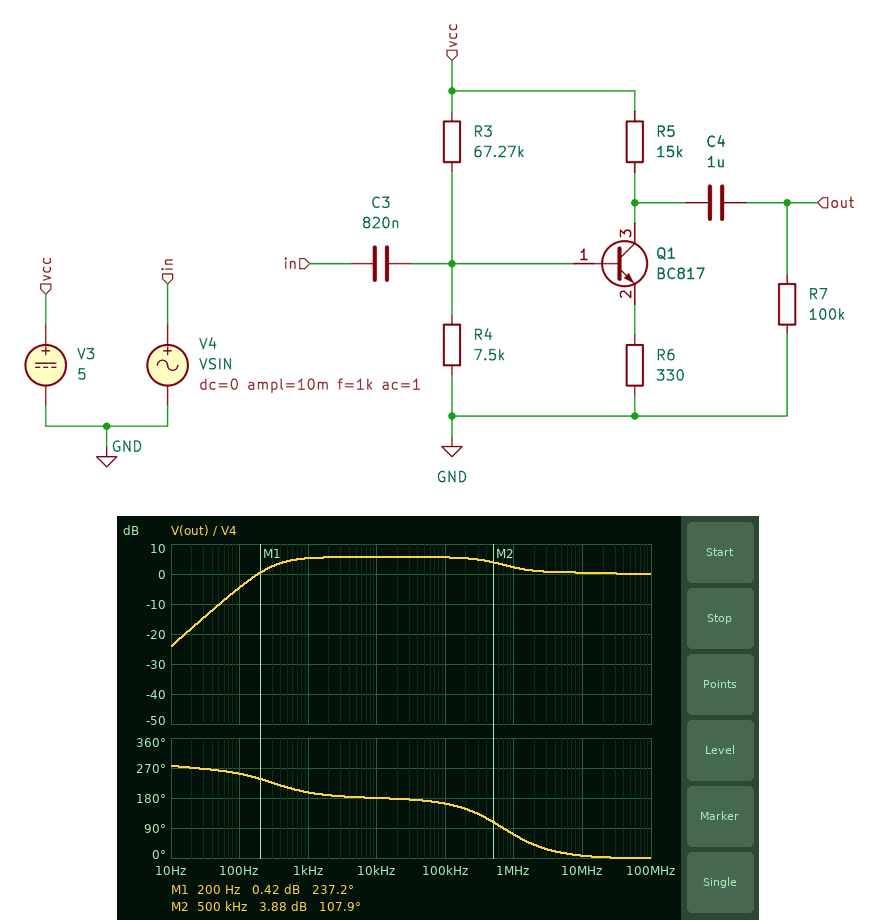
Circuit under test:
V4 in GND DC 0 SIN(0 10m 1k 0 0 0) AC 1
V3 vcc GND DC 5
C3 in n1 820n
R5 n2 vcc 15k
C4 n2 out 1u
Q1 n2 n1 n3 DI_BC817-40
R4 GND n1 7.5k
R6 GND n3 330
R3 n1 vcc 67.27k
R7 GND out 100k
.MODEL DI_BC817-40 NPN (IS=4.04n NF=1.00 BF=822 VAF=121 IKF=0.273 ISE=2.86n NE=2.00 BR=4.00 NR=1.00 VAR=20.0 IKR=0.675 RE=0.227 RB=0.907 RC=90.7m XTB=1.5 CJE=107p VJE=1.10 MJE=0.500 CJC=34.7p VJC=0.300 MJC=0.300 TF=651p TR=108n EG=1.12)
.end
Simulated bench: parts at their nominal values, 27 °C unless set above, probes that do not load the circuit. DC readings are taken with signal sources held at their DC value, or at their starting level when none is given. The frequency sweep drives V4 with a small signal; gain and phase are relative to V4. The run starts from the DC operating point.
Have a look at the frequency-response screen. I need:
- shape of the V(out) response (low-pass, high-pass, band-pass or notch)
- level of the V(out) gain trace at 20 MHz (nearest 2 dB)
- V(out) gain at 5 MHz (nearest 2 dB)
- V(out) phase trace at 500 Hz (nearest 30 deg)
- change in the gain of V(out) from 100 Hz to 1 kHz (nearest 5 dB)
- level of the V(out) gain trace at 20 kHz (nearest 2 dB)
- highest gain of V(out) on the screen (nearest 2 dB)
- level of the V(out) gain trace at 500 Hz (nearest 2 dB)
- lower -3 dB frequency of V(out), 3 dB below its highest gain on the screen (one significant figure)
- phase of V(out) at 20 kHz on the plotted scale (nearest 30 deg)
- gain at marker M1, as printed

high-pass
0 dB
0 dB
210 deg
10 dB
6 dB
6 dB
4 dB
300 Hz
180 deg
0.42 dB
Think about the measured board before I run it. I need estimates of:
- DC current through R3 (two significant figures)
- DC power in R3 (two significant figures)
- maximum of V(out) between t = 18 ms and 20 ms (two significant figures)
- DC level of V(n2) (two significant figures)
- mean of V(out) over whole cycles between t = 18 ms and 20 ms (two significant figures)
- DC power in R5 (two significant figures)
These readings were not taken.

68 µA
310 µW
59 mV
160 mV
9.6 mV
1.6 mW
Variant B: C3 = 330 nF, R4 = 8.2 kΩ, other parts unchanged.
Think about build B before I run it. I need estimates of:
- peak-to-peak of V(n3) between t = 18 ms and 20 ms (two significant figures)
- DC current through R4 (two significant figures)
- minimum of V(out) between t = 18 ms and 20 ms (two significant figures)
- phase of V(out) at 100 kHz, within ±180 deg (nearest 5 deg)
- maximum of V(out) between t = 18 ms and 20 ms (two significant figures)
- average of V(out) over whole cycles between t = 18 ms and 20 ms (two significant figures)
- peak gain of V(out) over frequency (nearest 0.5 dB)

8.3 mV
50 µA
-6.8 mV
160 deg
20 mV
2.9 mV
2.0 dB
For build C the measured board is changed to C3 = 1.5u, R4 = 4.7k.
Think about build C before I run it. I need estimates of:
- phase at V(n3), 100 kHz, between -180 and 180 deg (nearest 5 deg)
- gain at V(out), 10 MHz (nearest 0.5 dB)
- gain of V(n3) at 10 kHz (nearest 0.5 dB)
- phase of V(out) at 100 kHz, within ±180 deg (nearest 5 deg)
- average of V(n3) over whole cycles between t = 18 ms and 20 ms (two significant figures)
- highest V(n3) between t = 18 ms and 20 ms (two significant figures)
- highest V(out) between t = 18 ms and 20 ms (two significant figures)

0 deg
6.5 dB
-3.5 dB
170 deg
51 mV
57 mV
250 mV
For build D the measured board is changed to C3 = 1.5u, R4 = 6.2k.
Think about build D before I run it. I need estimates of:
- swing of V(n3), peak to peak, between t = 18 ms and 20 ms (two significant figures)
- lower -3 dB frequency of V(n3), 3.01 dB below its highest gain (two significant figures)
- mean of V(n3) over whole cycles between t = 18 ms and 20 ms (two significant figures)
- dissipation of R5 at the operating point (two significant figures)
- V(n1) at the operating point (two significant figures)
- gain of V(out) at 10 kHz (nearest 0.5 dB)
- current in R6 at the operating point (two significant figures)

13 mV
440 kHz
100 mV
1.5 mW
400 mV
19.0 dB
320 µA
